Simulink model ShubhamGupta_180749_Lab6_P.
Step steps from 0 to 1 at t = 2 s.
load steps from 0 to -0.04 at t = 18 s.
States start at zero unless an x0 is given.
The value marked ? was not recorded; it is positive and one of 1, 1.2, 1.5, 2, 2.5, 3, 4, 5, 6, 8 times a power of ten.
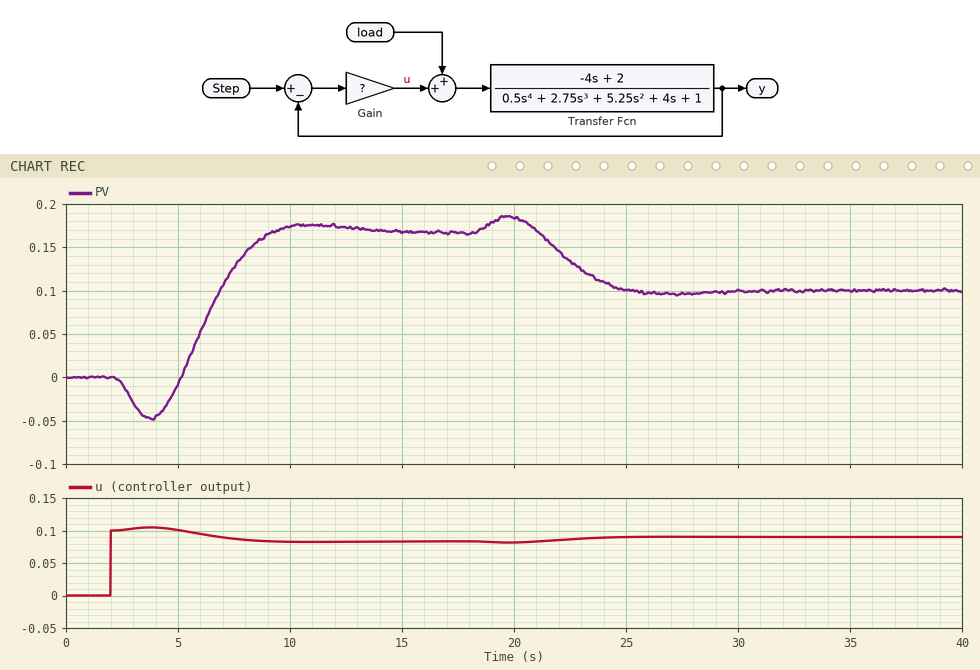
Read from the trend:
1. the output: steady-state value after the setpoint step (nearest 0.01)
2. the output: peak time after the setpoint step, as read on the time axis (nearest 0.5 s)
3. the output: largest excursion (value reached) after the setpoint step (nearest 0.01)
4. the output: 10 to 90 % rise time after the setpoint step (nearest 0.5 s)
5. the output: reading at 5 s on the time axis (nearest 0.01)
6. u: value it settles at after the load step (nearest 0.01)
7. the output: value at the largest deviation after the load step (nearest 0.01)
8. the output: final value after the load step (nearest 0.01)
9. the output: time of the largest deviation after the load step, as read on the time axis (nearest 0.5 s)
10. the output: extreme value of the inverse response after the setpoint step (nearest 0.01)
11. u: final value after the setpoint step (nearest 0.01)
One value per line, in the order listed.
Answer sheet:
0.17
11.0 s
0.18
3.0 s
-0.01
0.09
0.10
0.10
27.0 s
-0.05
0.08
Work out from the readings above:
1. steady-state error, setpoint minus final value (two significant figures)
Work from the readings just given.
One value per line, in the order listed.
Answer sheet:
0.83
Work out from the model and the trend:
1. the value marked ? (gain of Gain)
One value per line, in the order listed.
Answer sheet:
0.1
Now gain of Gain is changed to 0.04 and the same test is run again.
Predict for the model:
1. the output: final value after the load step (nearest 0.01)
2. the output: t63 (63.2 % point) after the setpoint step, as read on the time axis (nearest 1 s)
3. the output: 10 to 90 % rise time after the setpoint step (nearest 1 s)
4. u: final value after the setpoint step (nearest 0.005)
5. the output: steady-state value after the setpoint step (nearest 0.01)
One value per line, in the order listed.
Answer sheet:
0.00
7 s
4 s
0.035
0.07
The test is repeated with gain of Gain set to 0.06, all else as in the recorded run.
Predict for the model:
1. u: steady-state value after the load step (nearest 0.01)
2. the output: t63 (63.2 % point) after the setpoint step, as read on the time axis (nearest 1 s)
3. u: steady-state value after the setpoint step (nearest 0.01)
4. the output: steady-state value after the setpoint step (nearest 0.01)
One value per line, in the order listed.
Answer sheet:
0.06
7 s
0.05
0.11
